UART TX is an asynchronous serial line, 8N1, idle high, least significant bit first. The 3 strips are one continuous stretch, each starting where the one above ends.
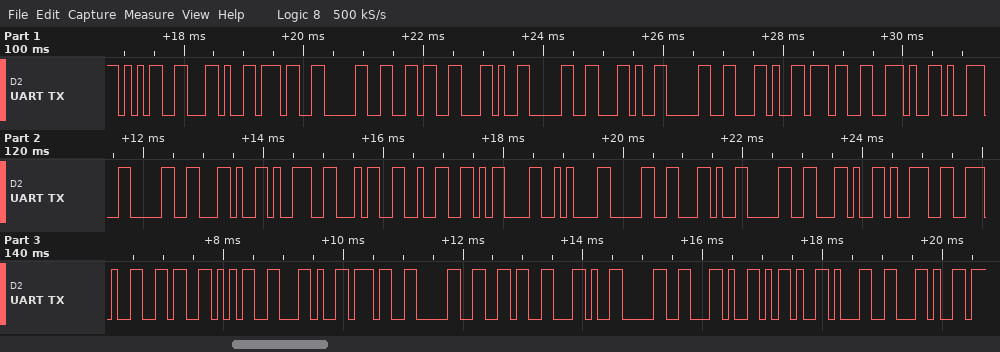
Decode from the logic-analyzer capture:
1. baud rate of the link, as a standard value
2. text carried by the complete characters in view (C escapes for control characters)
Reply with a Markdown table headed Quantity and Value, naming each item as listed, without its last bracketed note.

| Quantity | Value |
|---|---|
| baud rate of the link, as a standard value | 9600 baud |
| text carried by the complete characters in view | "5,706,0,0,7.90,942\r\n0,0,9.65,706,0,-1," |
